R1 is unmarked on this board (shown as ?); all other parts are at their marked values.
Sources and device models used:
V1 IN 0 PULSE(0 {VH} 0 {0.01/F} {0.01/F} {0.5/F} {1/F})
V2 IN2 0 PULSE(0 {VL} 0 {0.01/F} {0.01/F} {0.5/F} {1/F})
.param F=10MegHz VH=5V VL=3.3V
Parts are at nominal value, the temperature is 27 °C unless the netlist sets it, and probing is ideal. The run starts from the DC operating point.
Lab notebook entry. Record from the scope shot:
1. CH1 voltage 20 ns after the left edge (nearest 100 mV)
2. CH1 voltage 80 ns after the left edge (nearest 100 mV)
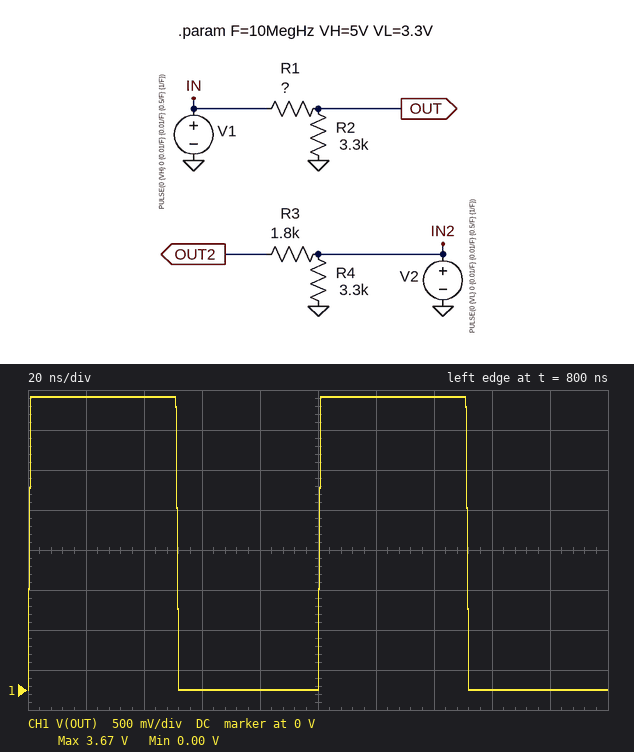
3.7 V
0 V
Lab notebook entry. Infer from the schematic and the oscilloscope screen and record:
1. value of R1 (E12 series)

1.2 kΩ
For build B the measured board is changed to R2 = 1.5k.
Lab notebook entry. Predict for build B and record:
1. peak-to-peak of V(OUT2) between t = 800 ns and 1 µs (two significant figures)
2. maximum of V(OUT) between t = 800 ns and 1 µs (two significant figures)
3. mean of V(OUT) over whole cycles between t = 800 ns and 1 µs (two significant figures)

3.3 V
2.8 V
1.4 V
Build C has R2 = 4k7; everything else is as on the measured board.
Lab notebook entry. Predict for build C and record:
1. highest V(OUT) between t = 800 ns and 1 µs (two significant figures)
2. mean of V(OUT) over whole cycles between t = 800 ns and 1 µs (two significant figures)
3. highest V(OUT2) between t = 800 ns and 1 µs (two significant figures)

4.0 V
2.0 V
3.3 V
